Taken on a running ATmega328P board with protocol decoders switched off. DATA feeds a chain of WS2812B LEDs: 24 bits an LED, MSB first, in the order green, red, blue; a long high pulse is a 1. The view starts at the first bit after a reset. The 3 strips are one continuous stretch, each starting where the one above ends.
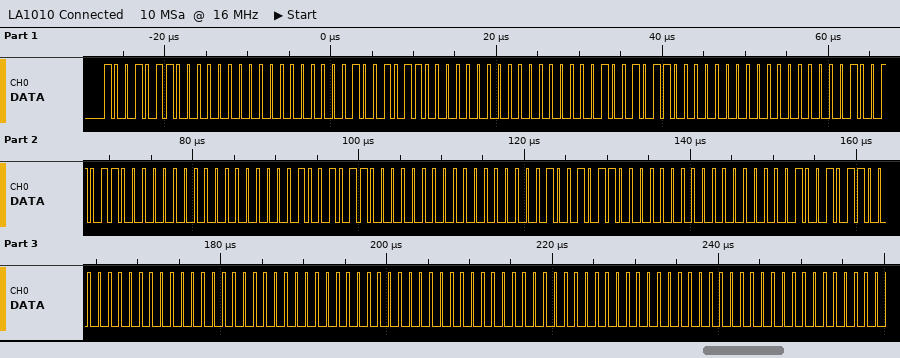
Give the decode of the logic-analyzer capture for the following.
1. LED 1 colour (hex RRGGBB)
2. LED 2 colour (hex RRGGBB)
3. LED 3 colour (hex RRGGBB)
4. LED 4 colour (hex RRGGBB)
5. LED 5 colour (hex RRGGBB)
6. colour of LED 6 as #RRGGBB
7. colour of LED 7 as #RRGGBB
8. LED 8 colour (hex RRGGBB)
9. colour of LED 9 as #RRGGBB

#009600
#009600
#009600
#009600
#009600
#009600
#009600
#000000
#000000
